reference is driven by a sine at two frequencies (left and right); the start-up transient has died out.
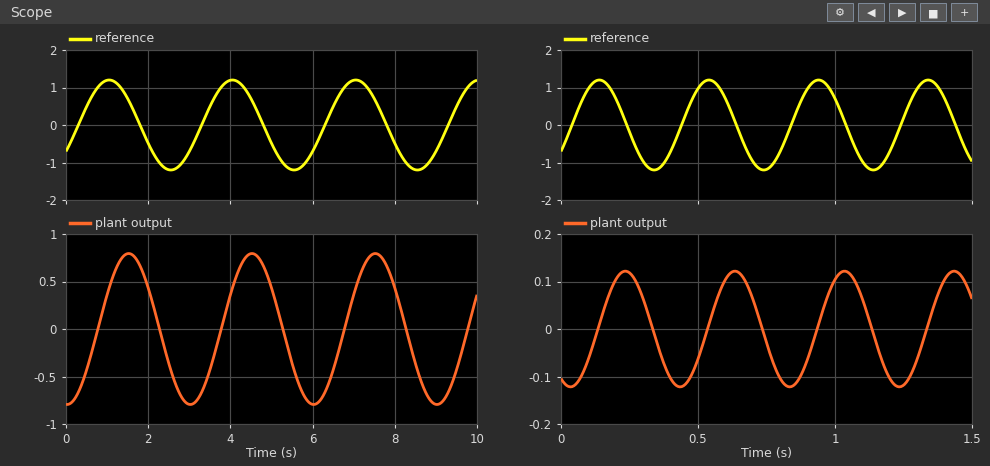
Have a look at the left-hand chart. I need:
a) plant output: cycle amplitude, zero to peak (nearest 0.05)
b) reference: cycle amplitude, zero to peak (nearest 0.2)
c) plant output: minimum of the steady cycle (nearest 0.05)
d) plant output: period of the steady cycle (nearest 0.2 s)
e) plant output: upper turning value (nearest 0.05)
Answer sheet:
0.80
1.2
-0.80
3.0 s
0.80
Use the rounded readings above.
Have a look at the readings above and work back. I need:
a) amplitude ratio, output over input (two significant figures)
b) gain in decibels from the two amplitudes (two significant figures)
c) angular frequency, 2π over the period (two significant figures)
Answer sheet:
0.67
-3.5 dB
2.1 rad/s
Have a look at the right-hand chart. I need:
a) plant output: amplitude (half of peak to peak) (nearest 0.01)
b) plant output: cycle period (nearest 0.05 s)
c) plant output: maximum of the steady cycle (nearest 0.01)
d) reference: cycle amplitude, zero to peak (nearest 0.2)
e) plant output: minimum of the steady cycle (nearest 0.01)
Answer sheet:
0.12
0.40 s
0.12
1.2
-0.12
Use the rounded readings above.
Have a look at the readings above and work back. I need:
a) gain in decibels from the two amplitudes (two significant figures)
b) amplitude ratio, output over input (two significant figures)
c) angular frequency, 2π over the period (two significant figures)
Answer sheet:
-20 dB
0.10
16 rad/s
